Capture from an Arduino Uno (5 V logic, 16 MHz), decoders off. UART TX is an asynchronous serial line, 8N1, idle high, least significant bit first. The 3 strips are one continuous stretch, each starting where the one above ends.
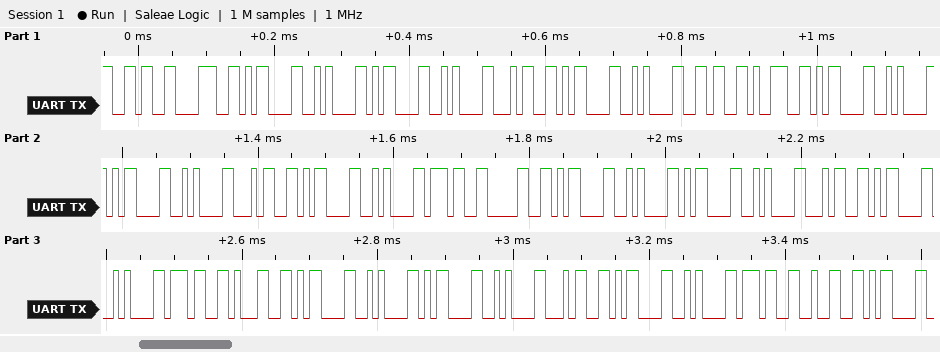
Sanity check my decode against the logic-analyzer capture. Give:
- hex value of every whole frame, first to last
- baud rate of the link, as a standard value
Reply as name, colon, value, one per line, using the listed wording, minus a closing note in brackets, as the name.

hex value of every whole frame, first to last: 36 38 0D 0A 0D 0A 34 0D 0A 36 39 0D 0A 0D 0A 34 0D 0A 37 30 0D 0A 0D 0A 34 0D 0A 37 31 0D 0A 0D 0A 34 0D 0A 37 32 0D
baud rate of the link, as a standard value: 115200 baud
